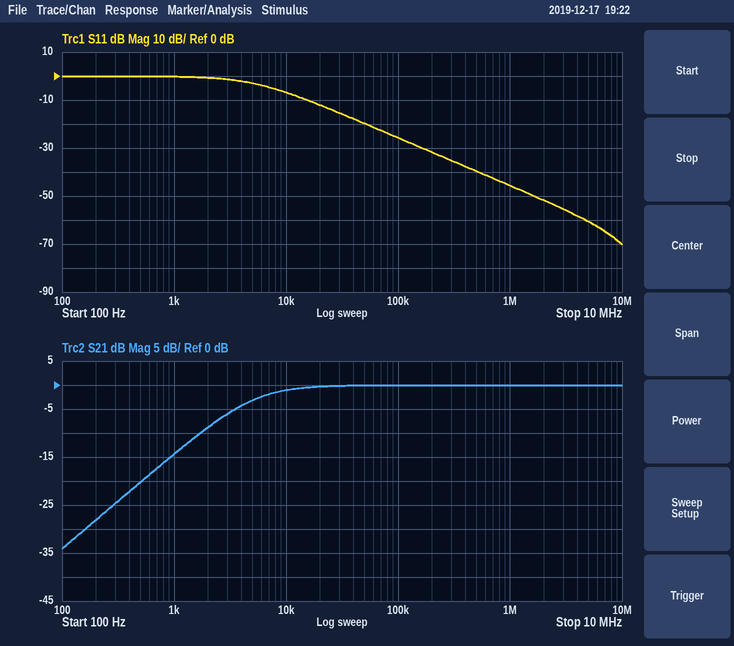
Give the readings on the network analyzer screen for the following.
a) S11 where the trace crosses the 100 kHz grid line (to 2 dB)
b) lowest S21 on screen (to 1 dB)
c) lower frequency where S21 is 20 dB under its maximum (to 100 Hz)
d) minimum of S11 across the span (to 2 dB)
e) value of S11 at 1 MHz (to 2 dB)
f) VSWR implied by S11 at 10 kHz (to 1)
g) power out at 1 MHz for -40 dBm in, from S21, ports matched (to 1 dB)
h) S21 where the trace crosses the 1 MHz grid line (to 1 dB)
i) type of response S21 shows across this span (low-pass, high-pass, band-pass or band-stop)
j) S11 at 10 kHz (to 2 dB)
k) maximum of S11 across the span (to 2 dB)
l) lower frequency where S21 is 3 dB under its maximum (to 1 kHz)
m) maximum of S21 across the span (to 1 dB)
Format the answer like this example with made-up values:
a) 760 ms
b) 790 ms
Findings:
a) -26 dB
b) -34 dB
c) 500 Hz
d) -70 dB
e) -46 dB
f) 3
g) -40 dBm
h) 0 dB
i) high-pass
j) -6 dB
k) 0 dB
l) 5 kHz
m) 0 dB
